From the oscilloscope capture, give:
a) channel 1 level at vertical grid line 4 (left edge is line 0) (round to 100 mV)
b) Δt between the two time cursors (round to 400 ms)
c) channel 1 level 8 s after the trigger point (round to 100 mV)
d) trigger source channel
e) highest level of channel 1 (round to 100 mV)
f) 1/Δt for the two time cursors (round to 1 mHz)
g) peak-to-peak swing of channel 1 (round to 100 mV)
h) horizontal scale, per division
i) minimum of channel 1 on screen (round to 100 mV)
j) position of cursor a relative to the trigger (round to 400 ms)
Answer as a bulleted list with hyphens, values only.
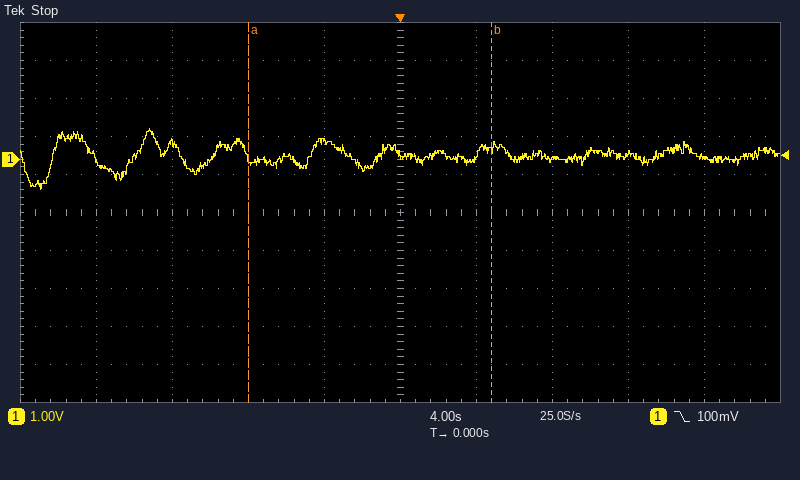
- 500 mV
- 12.8 s
- 0.0 V
- channel 1
- 800 mV
- 78 mHz
- 1.6 V
- 4 s
- -800 mV
- -8.0 s
